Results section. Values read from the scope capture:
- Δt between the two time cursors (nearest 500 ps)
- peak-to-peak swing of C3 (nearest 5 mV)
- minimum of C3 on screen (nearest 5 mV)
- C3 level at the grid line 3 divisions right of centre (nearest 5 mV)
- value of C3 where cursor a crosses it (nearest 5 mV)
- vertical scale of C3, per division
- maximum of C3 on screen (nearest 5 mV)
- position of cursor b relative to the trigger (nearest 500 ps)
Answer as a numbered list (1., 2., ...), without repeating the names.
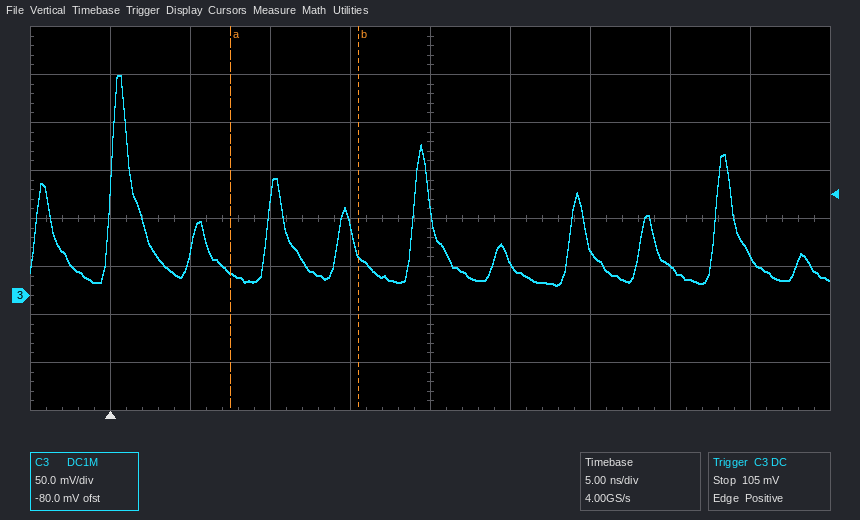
1. 8.0 ns
2. 220 mV
3. 10 mV
4. 30 mV
5. 25 mV
6. 50 mV
7. 230 mV
8. +15.5 ns
